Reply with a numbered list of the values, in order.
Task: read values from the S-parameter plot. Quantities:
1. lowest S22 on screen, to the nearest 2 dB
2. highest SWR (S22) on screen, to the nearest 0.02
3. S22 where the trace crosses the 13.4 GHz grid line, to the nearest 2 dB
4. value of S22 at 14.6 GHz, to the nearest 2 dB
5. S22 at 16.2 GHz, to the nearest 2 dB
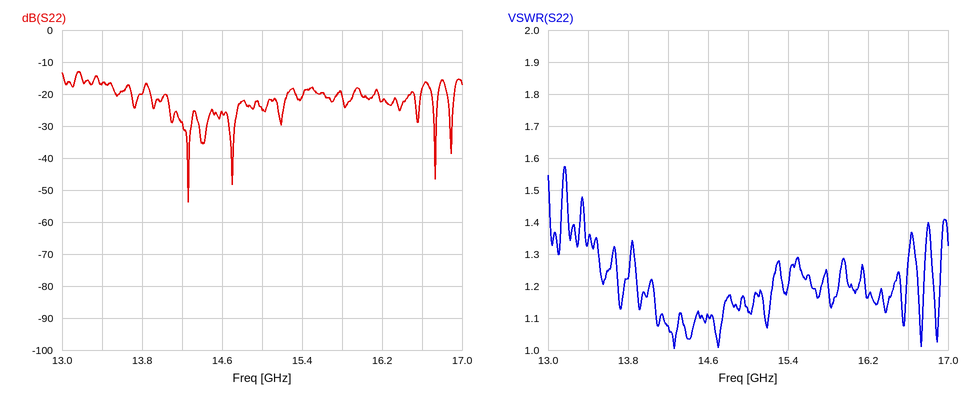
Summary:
1. -54 dB
2. 1.58
3. -16 dB
4. -26 dB
5. -22 dB
